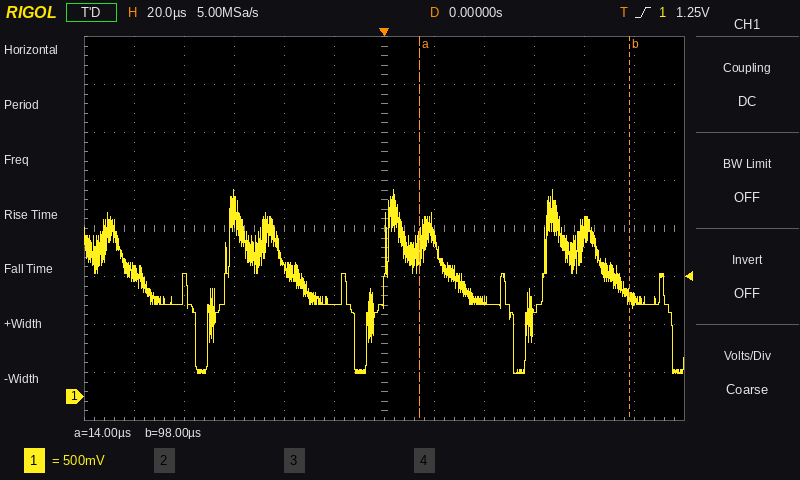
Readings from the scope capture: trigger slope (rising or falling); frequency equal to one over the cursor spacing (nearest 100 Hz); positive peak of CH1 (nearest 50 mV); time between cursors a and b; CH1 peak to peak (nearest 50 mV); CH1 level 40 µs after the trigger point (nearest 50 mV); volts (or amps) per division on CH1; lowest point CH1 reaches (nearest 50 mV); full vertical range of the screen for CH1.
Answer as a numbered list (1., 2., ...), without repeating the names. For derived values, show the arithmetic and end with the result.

1. rising
2. 1 / 84 µs ≈ 11.9 kHz
3. 2.15 V
4. 98 µs − (14 µs) = 84 µs
5. 2.15 V − (250 mV) = 1.90 V
6. 1.00 V
7. 500 mV
8. 250 mV
9. 4 V
